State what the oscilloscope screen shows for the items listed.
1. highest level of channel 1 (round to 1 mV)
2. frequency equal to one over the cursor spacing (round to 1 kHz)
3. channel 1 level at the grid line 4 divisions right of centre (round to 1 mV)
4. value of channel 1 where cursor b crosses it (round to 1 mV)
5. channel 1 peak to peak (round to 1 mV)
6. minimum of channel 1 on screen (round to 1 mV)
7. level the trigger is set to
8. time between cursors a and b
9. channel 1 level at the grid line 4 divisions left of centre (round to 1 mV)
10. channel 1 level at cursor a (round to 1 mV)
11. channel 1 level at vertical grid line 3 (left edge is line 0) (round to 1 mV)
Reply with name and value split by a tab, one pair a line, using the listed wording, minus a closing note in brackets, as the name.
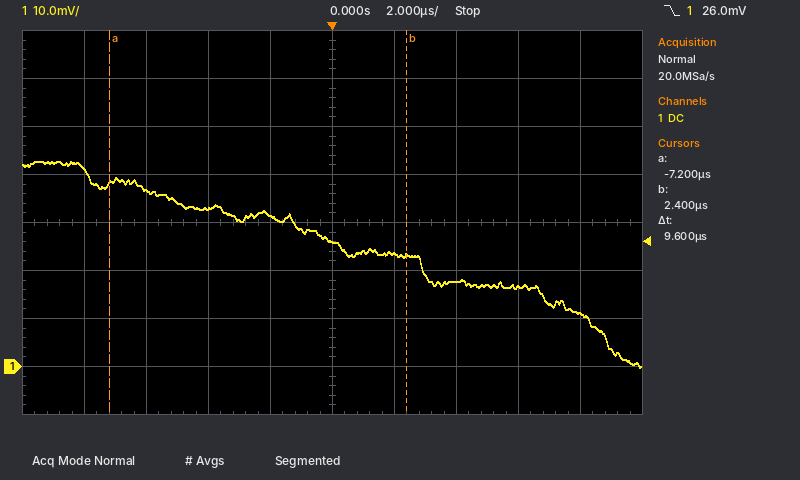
highest level of channel 1	43 mV
frequency equal to one over the cursor spacing	104 kHz
channel 1 level at the grid line 4 divisions right of centre	11 mV
value of channel 1 where cursor b crosses it	23 mV
channel 1 peak to peak	43 mV
minimum of channel 1 on screen	0 mV
level the trigger is set to	26.0 mV
time between cursors a and b	9.6 µs
channel 1 level at the grid line 4 divisions left of centre	41 mV
channel 1 level at cursor a	38 mV
channel 1 level at vertical grid line 3 (left edge is line 0)	33 mV
